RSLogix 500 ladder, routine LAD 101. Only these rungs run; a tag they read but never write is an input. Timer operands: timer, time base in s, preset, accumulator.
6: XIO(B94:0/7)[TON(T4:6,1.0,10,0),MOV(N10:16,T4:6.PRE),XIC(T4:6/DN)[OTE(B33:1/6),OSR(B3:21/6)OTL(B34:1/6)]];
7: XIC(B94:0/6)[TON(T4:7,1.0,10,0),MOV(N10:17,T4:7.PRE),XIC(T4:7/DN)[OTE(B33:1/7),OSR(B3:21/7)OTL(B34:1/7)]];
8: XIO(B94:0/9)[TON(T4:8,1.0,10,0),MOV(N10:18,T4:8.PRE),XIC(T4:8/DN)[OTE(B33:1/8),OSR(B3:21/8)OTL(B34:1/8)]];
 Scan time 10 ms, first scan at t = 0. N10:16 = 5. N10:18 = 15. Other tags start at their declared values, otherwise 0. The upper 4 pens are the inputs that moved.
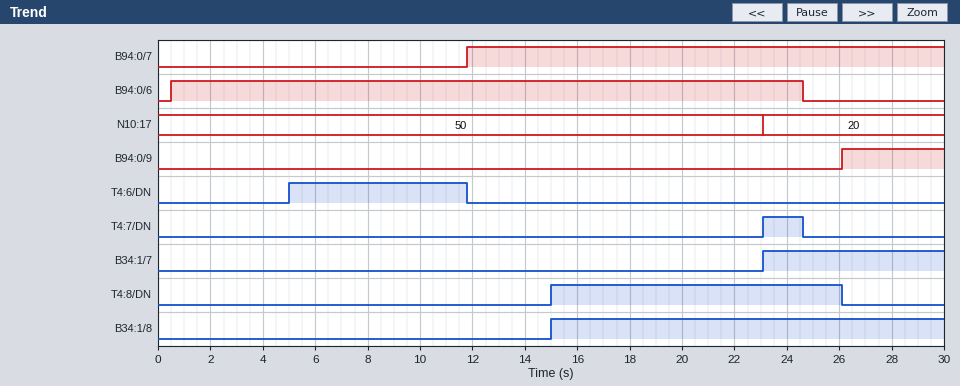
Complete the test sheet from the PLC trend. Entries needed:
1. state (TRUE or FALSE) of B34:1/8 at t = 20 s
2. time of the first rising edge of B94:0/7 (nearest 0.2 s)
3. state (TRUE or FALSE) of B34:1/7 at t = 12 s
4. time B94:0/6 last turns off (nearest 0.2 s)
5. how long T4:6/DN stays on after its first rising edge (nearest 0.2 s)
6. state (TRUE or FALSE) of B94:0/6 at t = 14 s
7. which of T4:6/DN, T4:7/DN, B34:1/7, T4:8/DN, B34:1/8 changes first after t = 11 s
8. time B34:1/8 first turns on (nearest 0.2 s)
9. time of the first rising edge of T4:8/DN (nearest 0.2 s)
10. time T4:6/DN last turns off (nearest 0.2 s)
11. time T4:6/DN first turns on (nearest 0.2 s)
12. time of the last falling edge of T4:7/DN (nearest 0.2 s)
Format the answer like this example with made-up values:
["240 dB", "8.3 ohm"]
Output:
["TRUE", "11.8 s", "FALSE", "24.6 s", "6.8 s", "TRUE", "T4:6/DN", "15.0 s", "15.0 s", "11.8 s", "5.0 s", "24.6 s"]
